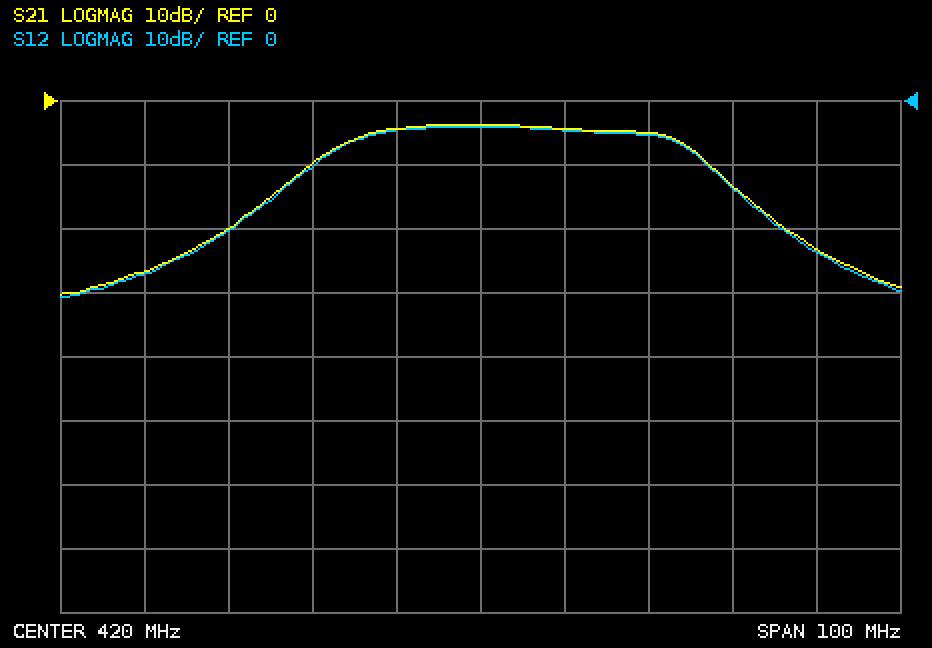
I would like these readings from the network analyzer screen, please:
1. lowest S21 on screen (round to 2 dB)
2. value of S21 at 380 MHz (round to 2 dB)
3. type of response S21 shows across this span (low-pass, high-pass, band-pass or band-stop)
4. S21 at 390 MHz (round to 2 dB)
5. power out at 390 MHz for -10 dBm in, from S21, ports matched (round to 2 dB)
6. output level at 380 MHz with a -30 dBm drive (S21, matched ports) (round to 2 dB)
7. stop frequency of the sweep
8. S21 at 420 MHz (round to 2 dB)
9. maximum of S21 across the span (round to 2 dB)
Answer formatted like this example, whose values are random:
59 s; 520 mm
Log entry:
-30 dB; -26 dB; band-pass; -20 dB; -30 dBm; -56 dBm; 470 MHz; -4 dB; -4 dB
